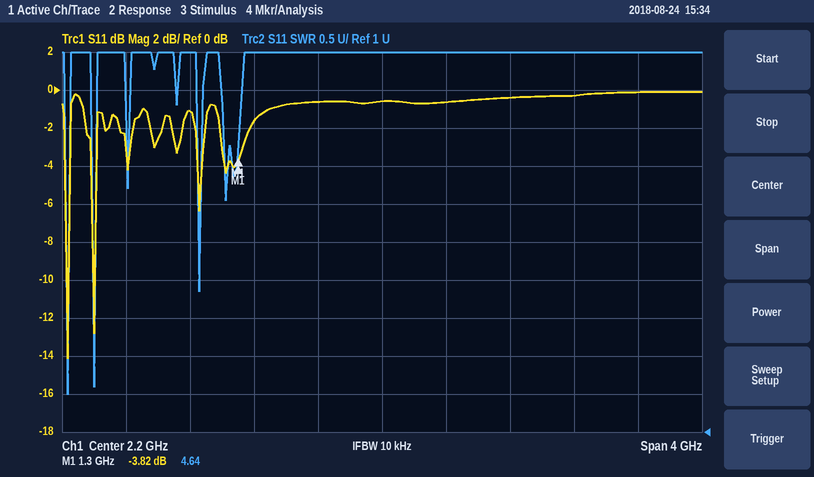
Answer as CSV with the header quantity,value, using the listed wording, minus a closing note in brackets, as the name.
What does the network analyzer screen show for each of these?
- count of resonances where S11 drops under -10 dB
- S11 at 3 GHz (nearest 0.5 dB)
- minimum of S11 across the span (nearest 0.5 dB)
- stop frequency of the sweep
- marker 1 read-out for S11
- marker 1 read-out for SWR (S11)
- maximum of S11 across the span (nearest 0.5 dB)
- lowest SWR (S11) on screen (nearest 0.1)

quantity,value
count of resonances where S11 drops under -10 dB,2
S11 at 3 GHz,-0.5 dB
minimum of S11 across the span,-14.0 dB
stop frequency of the sweep,4.2 GHz
marker 1 read-out for S11,-3.82 dB
marker 1 read-out for SWR,4.64
maximum of S11 across the span,0.0 dB
lowest SWR (S11) on screen,1.5
